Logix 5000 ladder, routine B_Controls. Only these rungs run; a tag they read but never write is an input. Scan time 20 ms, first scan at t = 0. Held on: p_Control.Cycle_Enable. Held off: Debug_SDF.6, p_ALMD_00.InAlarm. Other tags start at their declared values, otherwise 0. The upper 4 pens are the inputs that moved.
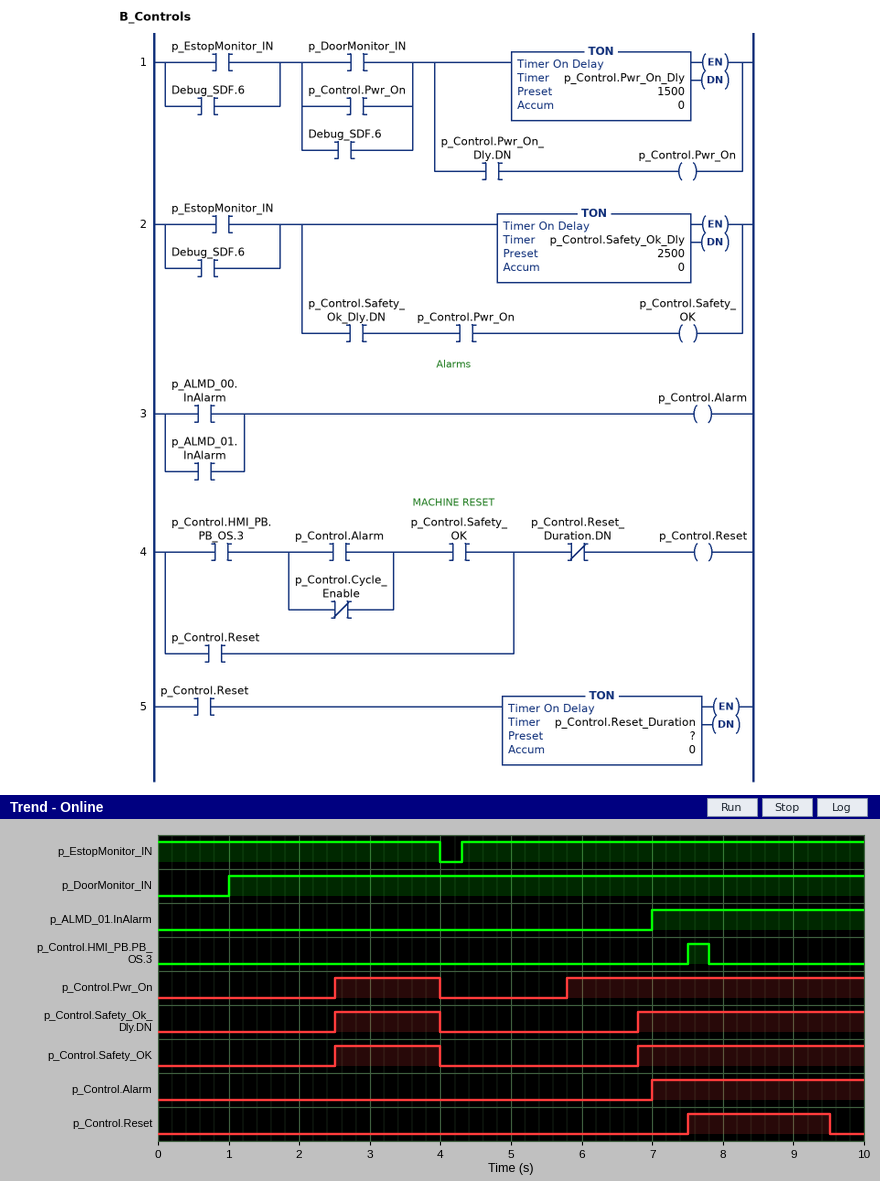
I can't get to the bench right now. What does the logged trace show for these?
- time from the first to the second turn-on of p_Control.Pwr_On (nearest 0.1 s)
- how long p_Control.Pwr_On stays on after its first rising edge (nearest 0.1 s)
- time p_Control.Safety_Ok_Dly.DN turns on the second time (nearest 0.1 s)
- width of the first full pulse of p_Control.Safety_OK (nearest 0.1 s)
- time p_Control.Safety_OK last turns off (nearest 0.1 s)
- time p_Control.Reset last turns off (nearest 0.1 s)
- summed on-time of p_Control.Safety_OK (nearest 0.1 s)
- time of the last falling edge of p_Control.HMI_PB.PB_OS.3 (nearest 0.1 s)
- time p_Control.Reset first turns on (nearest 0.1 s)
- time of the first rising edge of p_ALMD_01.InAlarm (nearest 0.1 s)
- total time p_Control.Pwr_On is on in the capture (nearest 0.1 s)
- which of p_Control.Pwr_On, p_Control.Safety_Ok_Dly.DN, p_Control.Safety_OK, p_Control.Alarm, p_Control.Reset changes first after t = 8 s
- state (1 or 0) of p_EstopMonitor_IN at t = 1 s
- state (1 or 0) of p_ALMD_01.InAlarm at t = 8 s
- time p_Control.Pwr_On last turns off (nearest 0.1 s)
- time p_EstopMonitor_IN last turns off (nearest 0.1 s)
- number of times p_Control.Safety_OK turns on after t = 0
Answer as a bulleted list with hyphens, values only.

- 3.3 s
- 1.5 s
- 6.8 s
- 1.5 s
- 4.0 s
- 9.5 s
- 4.7 s
- 7.8 s
- 7.5 s
- 7.0 s
- 5.7 s
- p_Control.Reset
- 1
- 1
- 4.0 s
- 4.0 s
- 2
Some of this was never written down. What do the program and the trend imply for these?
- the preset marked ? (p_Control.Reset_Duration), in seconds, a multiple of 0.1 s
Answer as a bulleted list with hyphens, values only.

- 2.0 s
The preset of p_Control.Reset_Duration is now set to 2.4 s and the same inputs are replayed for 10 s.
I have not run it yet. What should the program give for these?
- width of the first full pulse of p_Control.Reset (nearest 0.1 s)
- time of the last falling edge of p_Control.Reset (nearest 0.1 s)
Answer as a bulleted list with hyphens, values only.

- 2.4 s
- 9.9 s
